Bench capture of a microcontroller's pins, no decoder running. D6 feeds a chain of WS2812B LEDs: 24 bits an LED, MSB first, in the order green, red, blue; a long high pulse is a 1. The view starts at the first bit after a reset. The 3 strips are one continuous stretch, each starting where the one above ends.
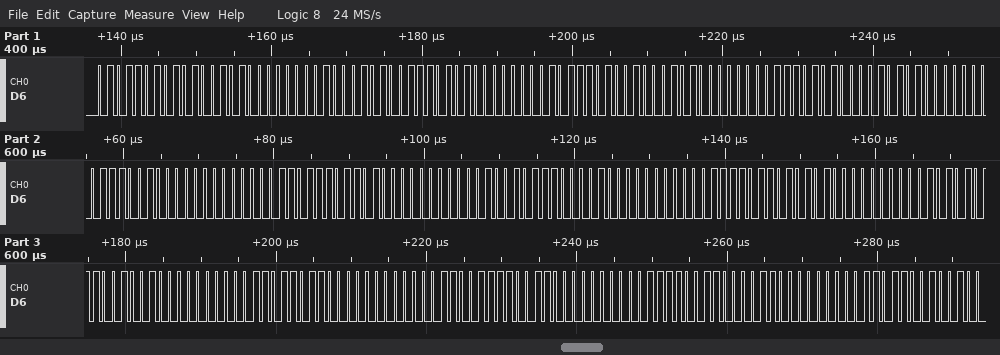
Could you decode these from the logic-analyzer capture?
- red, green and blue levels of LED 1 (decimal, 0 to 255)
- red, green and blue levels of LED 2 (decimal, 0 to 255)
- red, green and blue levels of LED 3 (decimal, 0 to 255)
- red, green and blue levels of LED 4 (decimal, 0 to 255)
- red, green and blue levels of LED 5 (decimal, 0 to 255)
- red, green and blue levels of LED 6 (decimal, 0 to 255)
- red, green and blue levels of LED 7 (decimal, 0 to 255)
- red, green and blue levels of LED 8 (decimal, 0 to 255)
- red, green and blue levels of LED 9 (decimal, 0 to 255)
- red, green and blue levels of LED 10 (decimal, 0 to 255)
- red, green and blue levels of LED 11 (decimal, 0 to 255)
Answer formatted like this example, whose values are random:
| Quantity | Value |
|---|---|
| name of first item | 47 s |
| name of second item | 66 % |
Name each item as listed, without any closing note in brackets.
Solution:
| Quantity | Value |
|---|---|
| red, green and blue levels of LED 1 | 165, 90, 0 |
| red, green and blue levels of LED 2 | 117, 138, 0 |
| red, green and blue levels of LED 3 | 69, 186, 0 |
| red, green and blue levels of LED 4 | 21, 234, 0 |
| red, green and blue levels of LED 5 | 0, 228, 27 |
| red, green and blue levels of LED 6 | 0, 180, 75 |
| red, green and blue levels of LED 7 | 0, 132, 123 |
| red, green and blue levels of LED 8 | 0, 84, 171 |
| red, green and blue levels of LED 9 | 0, 36, 219 |
| red, green and blue levels of LED 10 | 12, 0, 243 |
| red, green and blue levels of LED 11 | 60, 0, 195 |
